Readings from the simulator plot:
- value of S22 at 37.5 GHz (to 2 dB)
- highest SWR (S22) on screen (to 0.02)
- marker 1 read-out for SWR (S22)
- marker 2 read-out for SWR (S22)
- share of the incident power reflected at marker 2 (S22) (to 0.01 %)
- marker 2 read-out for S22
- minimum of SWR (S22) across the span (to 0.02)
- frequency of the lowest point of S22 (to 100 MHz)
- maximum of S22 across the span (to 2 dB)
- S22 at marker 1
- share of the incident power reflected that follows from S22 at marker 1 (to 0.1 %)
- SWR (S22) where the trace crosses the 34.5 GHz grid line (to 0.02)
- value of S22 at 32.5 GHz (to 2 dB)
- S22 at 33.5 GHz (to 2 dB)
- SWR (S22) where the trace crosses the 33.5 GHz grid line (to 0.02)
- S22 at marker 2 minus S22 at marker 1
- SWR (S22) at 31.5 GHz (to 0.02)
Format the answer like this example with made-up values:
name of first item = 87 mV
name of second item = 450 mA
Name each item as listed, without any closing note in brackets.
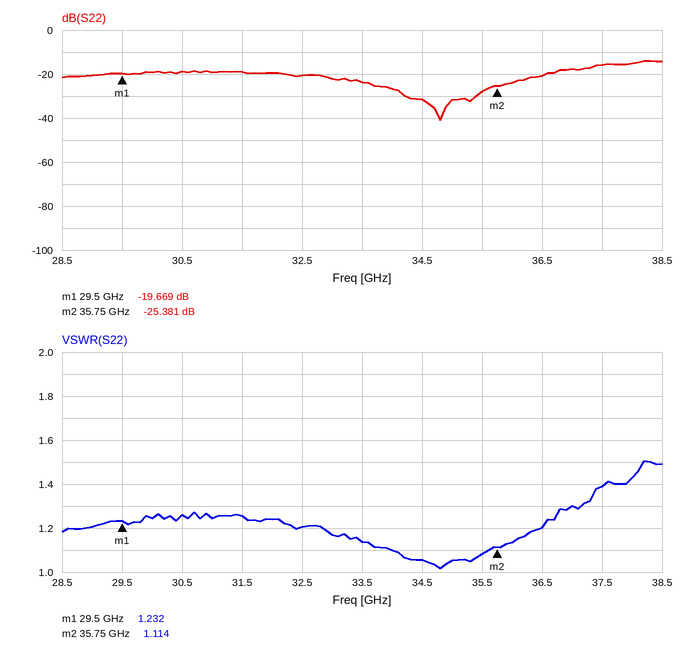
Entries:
value of S22 at 37.5 GHz = -16 dB
highest SWR (S22) on screen = 1.50
marker 1 read-out for SWR = 1.232
marker 2 read-out for SWR = 1.114
share of the incident power reflected at marker 2 (S22) = 0.29 %
marker 2 read-out for S22 = -25.381 dB
minimum of SWR (S22) across the span = 1.02
frequency of the lowest point of S22 = 34.8 GHz
maximum of S22 across the span = -14 dB
S22 at marker 1 = -19.669 dB
share of the incident power reflected that follows from S22 at marker 1 = 1.1 %
SWR (S22) where the trace crosses the 34.5 GHz grid line = 1.06
value of S22 at 32.5 GHz = -20 dB
S22 at 33.5 GHz = -24 dB
SWR (S22) where the trace crosses the 33.5 GHz grid line = 1.14
S22 at marker 2 minus S22 at marker 1 = -5.712 dB
SWR (S22) at 31.5 GHz = 1.26
